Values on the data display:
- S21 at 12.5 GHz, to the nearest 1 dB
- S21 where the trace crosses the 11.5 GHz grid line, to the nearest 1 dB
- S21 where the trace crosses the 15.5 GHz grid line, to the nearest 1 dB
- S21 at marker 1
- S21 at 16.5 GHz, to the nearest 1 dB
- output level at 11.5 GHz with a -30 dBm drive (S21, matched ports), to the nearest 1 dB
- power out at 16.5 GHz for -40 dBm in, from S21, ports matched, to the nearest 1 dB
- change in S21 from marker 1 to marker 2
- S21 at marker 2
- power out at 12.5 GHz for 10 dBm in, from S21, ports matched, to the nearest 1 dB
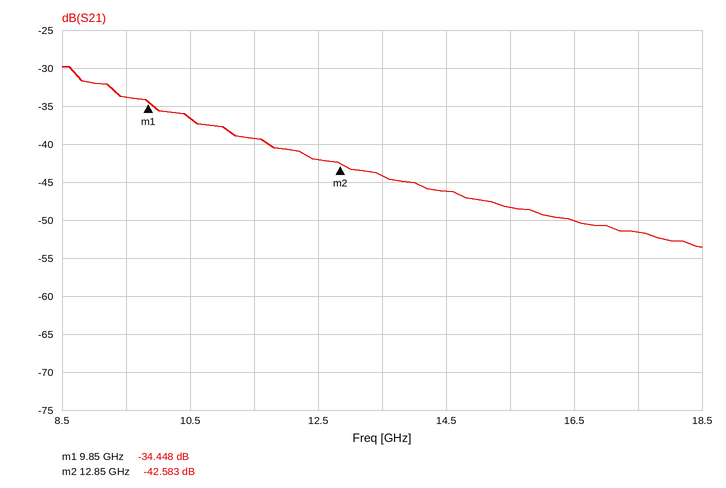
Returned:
-42 dB
-39 dB
-48 dB
-34.448 dB
-50 dB
-69 dBm
-90 dBm
-8.135 dB
-42.583 dB
-32 dBm
